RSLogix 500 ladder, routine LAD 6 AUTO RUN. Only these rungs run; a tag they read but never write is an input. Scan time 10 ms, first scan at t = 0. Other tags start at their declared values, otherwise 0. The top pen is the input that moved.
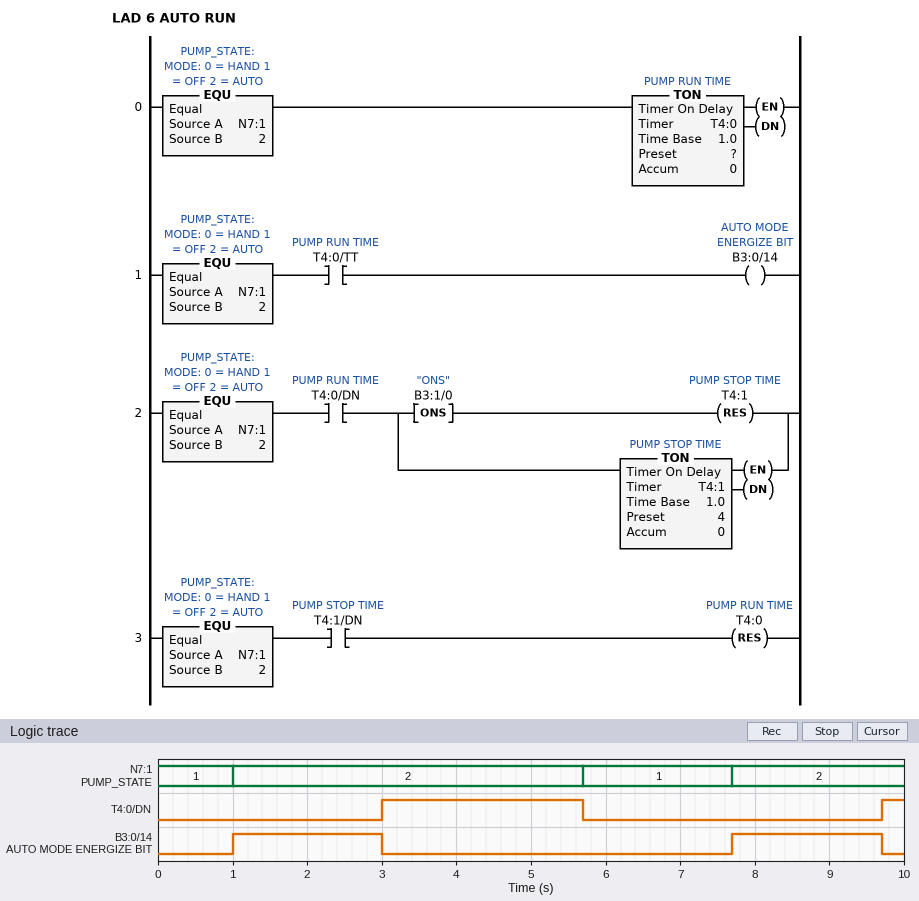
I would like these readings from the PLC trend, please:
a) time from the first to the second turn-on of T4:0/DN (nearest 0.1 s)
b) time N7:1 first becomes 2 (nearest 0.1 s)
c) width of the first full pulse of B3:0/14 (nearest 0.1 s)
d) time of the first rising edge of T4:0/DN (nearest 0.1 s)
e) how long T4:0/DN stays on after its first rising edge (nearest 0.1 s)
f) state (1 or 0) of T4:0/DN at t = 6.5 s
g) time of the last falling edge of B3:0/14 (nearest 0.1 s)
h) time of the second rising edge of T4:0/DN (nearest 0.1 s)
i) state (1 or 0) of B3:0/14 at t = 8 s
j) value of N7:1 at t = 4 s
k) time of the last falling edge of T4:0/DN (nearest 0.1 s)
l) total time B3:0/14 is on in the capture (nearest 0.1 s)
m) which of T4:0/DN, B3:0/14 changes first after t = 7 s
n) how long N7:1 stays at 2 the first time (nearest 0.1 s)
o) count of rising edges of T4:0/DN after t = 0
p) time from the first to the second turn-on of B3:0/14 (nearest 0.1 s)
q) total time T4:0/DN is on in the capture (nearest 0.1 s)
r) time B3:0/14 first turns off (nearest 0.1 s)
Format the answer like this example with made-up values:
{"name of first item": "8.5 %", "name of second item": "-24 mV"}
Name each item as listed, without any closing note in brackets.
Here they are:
{"time from the first to the second turn-on of T4:0/DN": "6.7 s", "time N7:1 first becomes 2": "1.0 s", "width of the first full pulse of B3:0/14": "2.0 s", "time of the first rising edge of T4:0/DN": "3.0 s", "how long T4:0/DN stays on after its first rising edge": "2.7 s", "state (1 or 0) of T4:0/DN at t = 6.5 s": "0", "time of the last falling edge of B3:0/14": "9.7 s", "time of the second rising edge of T4:0/DN": "9.7 s", "state (1 or 0) of B3:0/14 at t = 8 s": "1", "value of N7:1 at t = 4 s": "2", "time of the last falling edge of T4:0/DN": "5.7 s", "total time B3:0/14 is on in the capture": "4.0 s", "which of T4:0/DN, B3:0/14 changes first after t = 7 s": "B3:0/14", "how long N7:1 stays at 2 the first time": "4.7 s", "count of rising edges of T4:0/DN after t = 0": "2", "time from the first to the second turn-on of B3:0/14": "6.7 s", "total time T4:0/DN is on in the capture": "3.0 s", "time B3:0/14 first turns off": "3.0 s"}
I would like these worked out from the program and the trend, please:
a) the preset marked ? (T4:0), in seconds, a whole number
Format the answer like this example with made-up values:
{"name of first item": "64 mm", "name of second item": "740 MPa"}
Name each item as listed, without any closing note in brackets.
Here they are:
{"the preset marked ? (T4:0), in seconds, a whole number": "2 s"}
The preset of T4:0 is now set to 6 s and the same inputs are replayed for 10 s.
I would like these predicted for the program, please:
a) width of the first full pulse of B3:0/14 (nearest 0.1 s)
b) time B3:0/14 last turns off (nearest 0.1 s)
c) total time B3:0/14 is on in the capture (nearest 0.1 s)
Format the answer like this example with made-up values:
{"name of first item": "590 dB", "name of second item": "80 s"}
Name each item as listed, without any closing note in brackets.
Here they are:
{"width of the first full pulse of B3:0/14": "4.7 s", "time B3:0/14 last turns off": "5.7 s", "total time B3:0/14 is on in the capture": "7.0 s"}
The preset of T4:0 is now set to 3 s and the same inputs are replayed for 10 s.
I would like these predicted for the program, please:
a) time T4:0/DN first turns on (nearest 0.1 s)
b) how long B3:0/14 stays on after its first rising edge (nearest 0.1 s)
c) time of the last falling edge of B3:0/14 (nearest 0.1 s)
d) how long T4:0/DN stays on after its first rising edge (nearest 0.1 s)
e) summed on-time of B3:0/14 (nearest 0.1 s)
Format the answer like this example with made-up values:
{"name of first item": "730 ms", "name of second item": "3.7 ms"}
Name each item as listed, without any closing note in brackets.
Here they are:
{"time T4:0/DN first turns on": "4.0 s", "how long B3:0/14 stays on after its first rising edge": "3.0 s", "time of the last falling edge of B3:0/14": "4.0 s", "how long T4:0/DN stays on after its first rising edge": "1.7 s", "summed on-time of B3:0/14": "5.3 s"}
